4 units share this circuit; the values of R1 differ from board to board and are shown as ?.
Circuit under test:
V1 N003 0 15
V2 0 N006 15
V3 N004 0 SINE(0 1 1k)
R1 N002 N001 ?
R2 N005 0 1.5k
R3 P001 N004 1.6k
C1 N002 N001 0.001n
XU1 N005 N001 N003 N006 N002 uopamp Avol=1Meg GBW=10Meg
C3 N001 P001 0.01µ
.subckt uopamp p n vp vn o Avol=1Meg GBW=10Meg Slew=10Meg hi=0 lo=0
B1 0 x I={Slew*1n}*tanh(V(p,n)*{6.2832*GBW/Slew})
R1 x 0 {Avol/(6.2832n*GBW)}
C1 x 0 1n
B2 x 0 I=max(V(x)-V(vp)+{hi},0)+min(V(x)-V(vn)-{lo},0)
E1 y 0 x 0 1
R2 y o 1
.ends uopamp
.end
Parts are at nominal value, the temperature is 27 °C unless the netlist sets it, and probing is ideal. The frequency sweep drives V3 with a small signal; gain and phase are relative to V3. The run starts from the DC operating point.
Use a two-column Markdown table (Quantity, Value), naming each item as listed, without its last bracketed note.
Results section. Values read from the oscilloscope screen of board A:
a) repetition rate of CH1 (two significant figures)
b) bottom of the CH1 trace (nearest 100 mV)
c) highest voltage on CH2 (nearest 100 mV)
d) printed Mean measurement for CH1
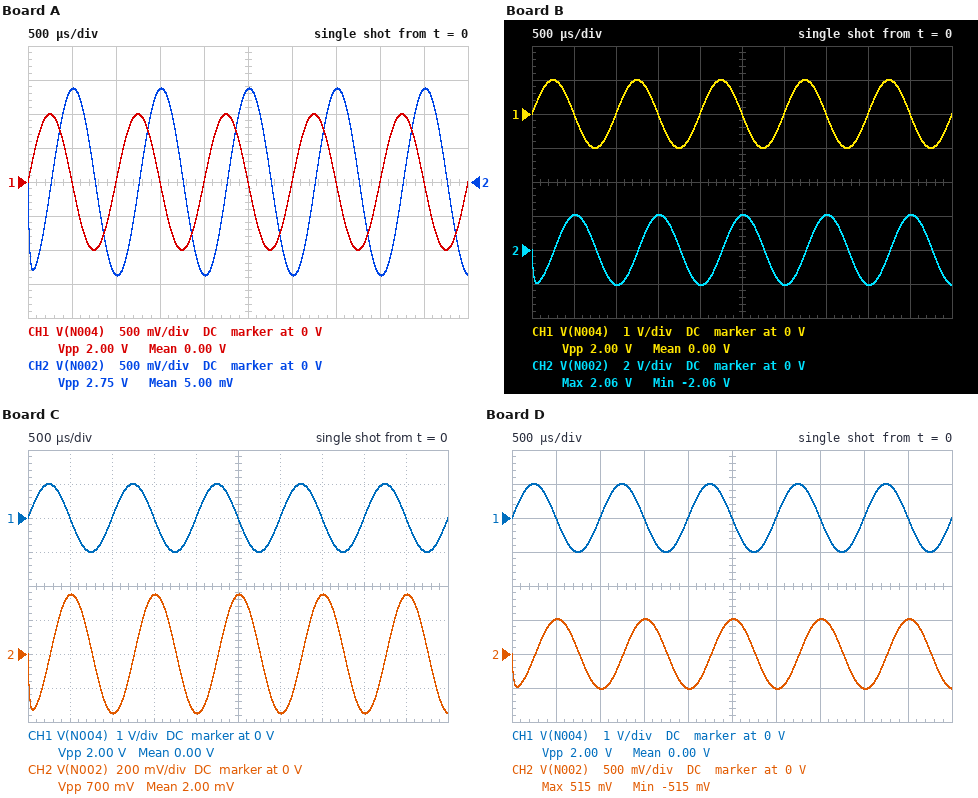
| Quantity | Value |
|---|---|
| repetition rate of CH1 | 1.0 kHz |
| bottom of the CH1 trace | -1.0 V |
| highest voltage on CH2 | 1.4 V |
| printed Mean measurement for CH1 | 0.00 V |
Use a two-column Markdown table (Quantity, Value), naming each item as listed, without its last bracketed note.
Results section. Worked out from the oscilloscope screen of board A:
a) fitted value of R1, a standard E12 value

| Quantity | Value |
|---|---|
| fitted value of R1, a standard E12 value | 22 kΩ |
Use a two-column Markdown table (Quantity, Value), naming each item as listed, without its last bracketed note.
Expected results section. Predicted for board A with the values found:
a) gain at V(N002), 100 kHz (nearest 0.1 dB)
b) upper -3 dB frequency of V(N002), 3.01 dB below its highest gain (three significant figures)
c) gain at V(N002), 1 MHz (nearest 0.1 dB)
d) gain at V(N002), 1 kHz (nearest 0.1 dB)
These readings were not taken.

| Quantity | Value |
|---|---|
| gain at V(N002), 100 kHz | 22.7 dB |
| upper -3 dB frequency of V(N002), 3.01 dB below its highest gain | 634 kHz |
| gain at V(N002), 1 MHz | 17.3 dB |
| gain at V(N002), 1 kHz | 2.8 dB |
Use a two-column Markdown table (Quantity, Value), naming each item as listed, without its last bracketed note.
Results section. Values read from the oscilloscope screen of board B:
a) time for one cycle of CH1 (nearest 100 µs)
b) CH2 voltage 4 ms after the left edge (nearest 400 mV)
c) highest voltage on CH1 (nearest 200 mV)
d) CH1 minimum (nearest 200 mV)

| Quantity | Value |
|---|---|
| time for one cycle of CH1 | 1.0 ms |
| CH2 voltage 4 ms after the left edge | -2.0 V |
| highest voltage on CH1 | 1.0 V |
| CH1 minimum | -1.0 V |
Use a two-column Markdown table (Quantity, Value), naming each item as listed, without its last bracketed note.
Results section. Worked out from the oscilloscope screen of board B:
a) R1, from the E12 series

| Quantity | Value |
|---|---|
| R1, from the E12 series | 33 kΩ |
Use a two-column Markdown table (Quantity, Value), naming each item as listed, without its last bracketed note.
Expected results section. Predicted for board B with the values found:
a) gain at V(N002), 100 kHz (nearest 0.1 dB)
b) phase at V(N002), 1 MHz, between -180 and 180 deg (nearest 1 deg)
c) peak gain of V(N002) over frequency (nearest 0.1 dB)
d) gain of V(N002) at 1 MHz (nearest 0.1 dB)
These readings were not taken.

| Quantity | Value |
|---|---|
| gain at V(N002), 100 kHz | 26.2 dB |
| phase at V(N002), 1 MHz, between -180 and 180 deg | 113 deg |
| peak gain of V(N002) over frequency | 26.3 dB |
| gain of V(N002) at 1 MHz | 18.1 dB |
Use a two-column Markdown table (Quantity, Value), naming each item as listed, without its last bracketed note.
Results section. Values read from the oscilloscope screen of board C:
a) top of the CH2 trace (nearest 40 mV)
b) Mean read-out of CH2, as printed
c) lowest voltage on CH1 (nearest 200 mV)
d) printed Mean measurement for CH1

| Quantity | Value |
|---|---|
| top of the CH2 trace | 360 mV |
| Mean read-out of CH2, as printed | 2.00 mV |
| lowest voltage on CH1 | -1.0 V |
| printed Mean measurement for CH1 | 0.00 V |
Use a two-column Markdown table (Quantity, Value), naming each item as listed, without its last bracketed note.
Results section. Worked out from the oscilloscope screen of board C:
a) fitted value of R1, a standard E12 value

| Quantity | Value |
|---|---|
| fitted value of R1, a standard E12 value | 5.6 kΩ |
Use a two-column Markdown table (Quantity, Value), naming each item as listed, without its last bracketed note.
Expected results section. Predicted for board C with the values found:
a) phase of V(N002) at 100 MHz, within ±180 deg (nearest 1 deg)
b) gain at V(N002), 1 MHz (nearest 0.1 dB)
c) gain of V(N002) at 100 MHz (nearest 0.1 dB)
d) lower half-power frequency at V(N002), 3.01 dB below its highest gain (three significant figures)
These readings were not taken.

| Quantity | Value |
|---|---|
| phase of V(N002) at 100 MHz, within ±180 deg | 55 deg |
| gain at V(N002), 1 MHz | 10.0 dB |
| gain of V(N002) at 100 MHz | -24.5 dB |
| lower half-power frequency at V(N002), 3.01 dB below its highest gain | 9.89 kHz |
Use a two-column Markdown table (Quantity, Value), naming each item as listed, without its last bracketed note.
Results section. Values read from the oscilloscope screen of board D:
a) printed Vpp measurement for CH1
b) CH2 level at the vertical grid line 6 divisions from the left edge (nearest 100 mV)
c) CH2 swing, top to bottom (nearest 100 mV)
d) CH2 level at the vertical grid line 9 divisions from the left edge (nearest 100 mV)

| Quantity | Value |
|---|---|
| printed Vpp measurement for CH1 | 2.00 V |
| CH2 level at the vertical grid line 6 divisions from the left edge | -500 mV |
| CH2 swing, top to bottom | 1.0 V |
| CH2 level at the vertical grid line 9 divisions from the left edge | 500 mV |
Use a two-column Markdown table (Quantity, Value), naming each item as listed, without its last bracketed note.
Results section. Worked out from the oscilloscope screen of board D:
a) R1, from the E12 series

| Quantity | Value |
|---|---|
| R1, from the E12 series | 8.2 kΩ |
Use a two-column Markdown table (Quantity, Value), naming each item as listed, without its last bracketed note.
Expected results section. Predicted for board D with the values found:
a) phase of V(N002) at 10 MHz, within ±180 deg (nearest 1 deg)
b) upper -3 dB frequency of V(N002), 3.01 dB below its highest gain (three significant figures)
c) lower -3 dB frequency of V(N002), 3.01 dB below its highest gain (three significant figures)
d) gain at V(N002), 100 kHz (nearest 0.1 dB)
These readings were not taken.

| Quantity | Value |
|---|---|
| phase of V(N002) at 10 MHz, within ±180 deg | 94 deg |
| upper -3 dB frequency of V(N002), 3.01 dB below its highest gain | 1.54 MHz |
| lower -3 dB frequency of V(N002), 3.01 dB below its highest gain | 9.87 kHz |
| gain at V(N002), 100 kHz | 14.2 dB |
